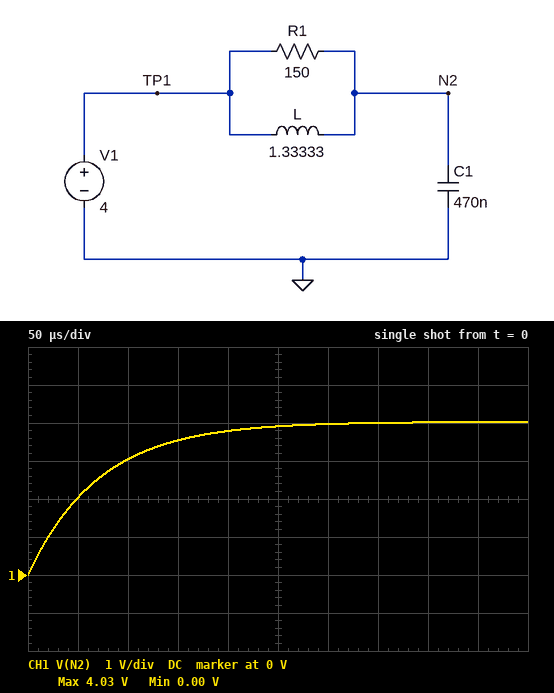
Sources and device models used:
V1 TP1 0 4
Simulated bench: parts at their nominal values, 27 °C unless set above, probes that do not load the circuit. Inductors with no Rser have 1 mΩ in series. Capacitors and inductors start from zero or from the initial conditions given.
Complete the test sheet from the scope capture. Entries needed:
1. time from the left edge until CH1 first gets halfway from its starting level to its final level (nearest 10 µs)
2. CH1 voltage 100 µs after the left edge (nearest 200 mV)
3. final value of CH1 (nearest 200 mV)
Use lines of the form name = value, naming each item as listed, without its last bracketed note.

time from the left edge until CH1 first gets halfway from its starting level to its final level = 50 µs
CH1 voltage 100 µs after the left edge = 3.0 V
final value of CH1 = 4.0 V
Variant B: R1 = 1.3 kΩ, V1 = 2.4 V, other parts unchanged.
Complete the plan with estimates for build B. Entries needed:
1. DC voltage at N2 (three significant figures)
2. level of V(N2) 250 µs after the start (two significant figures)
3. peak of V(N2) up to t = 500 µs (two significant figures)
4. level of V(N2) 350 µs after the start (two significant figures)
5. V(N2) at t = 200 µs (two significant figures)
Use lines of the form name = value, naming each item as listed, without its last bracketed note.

DC voltage at N2 = 2.40 V
level of V(N2) 250 µs after the start = 900 mV
peak of V(N2) up to t = 500 µs = 1.6 V
level of V(N2) 350 µs after the start = 1.2 V
V(N2) at t = 200 µs = 730 mV
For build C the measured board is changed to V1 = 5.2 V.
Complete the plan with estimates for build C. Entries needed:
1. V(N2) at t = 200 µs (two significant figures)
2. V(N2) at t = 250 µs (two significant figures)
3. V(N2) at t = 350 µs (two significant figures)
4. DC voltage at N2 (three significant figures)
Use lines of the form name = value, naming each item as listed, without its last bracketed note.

V(N2) at t = 200 µs = 4.9 V
V(N2) at t = 250 µs = 5.1 V
V(N2) at t = 350 µs = 5.2 V
DC voltage at N2 = 5.20 V
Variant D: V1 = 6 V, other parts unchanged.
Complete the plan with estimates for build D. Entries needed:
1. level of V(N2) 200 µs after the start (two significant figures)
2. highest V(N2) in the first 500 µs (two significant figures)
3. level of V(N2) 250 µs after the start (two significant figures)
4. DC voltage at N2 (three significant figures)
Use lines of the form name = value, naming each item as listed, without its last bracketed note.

level of V(N2) 200 µs after the start = 5.7 V
highest V(N2) in the first 500 µs = 6.0 V
level of V(N2) 250 µs after the start = 5.9 V
DC voltage at N2 = 6.00 V
